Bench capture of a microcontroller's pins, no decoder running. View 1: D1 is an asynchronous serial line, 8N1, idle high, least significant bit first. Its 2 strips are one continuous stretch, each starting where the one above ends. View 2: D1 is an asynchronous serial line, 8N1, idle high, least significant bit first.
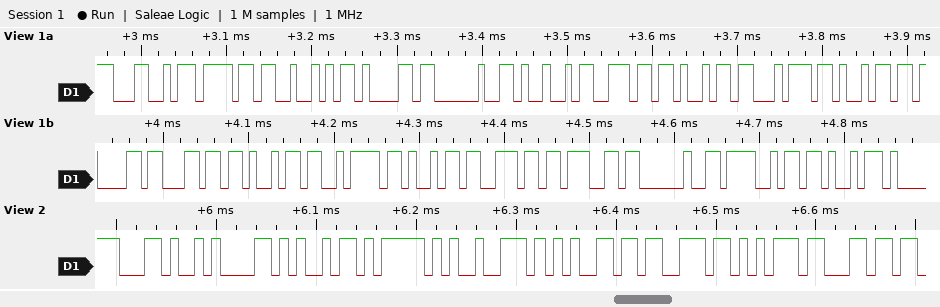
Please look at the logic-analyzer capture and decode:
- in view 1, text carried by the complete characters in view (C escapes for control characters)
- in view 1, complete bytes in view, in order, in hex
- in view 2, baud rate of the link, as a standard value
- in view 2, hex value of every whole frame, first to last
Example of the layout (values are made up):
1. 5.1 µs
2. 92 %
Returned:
1. "LoRa Initializing OK"
2. 4C 6F 52 61 20 49 6E 69 74 69 61 6C 69 7A 69 6E 67 20 4F 4B
3. 115200 baud
4. 2C 61 69 5F 72 65 73 75 6C
